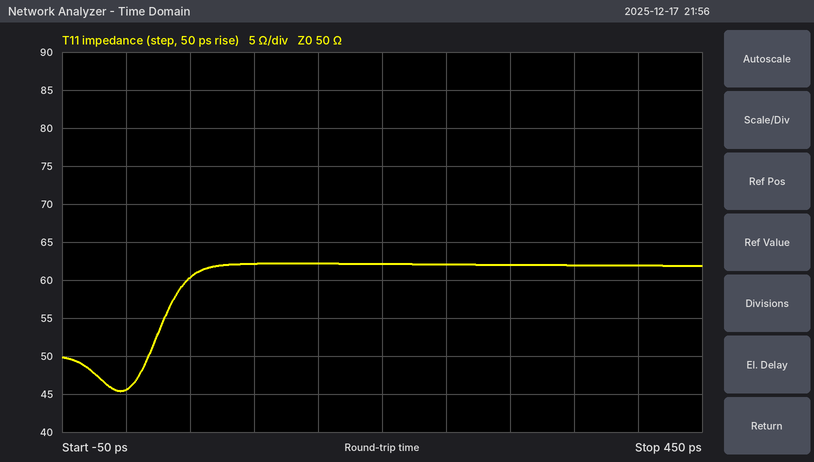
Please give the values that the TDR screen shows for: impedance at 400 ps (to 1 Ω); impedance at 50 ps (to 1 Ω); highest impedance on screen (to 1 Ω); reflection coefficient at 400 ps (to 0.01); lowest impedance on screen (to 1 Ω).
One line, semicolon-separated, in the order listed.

62 Ω; 60 Ω; 62 Ω; +0.11; 45 Ω
